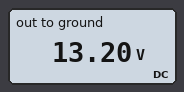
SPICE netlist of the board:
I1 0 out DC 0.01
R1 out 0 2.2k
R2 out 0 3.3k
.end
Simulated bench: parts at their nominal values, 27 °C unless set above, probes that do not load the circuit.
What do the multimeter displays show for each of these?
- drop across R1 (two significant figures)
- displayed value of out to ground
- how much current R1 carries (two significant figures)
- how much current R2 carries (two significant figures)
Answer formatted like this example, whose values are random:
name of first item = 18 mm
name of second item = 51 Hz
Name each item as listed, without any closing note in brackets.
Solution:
drop across R1 = 13 V
displayed value of out to ground = 13.20 V
how much current R1 carries = 6.0 mA
how much current R2 carries = 4.0 mA
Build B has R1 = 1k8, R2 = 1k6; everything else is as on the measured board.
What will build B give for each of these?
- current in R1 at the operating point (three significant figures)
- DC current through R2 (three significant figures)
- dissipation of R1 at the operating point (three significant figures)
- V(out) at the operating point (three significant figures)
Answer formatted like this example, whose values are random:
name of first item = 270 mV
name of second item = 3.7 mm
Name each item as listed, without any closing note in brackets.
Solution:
current in R1 at the operating point = 4.71 mA
DC current through R2 = 5.29 mA
dissipation of R1 at the operating point = 39.9 mW
V(out) at the operating point = 8.47 V
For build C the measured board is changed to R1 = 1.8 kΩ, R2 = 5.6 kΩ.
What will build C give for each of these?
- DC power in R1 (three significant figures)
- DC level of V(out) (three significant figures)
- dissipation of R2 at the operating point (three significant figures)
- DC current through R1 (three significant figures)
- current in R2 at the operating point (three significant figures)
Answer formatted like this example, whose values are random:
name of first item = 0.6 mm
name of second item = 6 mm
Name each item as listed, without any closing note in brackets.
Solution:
DC power in R1 = 103 mW
DC level of V(out) = 13.6 V
dissipation of R2 at the operating point = 33.1 mW
DC current through R1 = 7.57 mA
current in R2 at the operating point = 2.43 mA
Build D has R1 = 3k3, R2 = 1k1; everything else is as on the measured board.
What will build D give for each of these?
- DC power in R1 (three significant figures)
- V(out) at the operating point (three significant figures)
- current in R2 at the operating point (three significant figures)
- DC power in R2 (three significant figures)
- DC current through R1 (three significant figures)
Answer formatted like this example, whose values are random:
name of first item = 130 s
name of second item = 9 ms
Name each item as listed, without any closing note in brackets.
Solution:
DC power in R1 = 20.6 mW
V(out) at the operating point = 8.25 V
current in R2 at the operating point = 7.50 mA
DC power in R2 = 61.9 mW
DC current through R1 = 2.50 mA
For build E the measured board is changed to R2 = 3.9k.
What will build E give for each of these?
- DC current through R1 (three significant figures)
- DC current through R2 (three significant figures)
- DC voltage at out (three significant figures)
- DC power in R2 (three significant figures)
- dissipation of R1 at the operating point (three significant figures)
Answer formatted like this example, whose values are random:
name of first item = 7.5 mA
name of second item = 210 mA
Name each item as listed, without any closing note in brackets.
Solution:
DC current through R1 = 6.39 mA
DC current through R2 = 3.61 mA
DC voltage at out = 14.1 V
DC power in R2 = 50.7 mW
dissipation of R1 at the operating point = 89.9 mW
